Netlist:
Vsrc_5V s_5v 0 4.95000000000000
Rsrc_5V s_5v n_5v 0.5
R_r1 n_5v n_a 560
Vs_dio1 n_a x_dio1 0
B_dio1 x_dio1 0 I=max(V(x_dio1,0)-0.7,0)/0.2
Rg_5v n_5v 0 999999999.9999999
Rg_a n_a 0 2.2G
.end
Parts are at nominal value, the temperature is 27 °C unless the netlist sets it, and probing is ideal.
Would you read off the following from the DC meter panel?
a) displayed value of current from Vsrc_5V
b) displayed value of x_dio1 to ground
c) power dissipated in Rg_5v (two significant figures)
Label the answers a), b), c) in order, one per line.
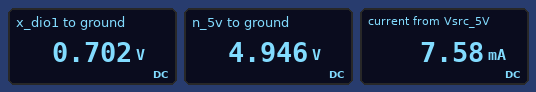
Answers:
a) 7.58 mA
b) 0.702 V
c) 24 nW
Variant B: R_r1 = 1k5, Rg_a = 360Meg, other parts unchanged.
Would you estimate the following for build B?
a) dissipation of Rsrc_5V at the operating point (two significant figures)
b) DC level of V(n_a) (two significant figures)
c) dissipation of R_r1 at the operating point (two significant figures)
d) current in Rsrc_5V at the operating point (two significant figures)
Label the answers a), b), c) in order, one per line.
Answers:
a) 4.0 µW
b) 700 mV
c) 12 mW
d) 2.8 mA
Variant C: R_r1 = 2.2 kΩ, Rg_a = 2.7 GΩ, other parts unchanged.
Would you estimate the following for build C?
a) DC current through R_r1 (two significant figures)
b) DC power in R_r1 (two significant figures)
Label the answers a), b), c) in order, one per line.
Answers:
a) 1.9 mA
b) 8.2 mW
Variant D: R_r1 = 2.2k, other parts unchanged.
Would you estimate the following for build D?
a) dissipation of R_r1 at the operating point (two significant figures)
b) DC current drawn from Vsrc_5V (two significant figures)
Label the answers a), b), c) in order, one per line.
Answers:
a) 8.2 mW
b) 1.9 mA
